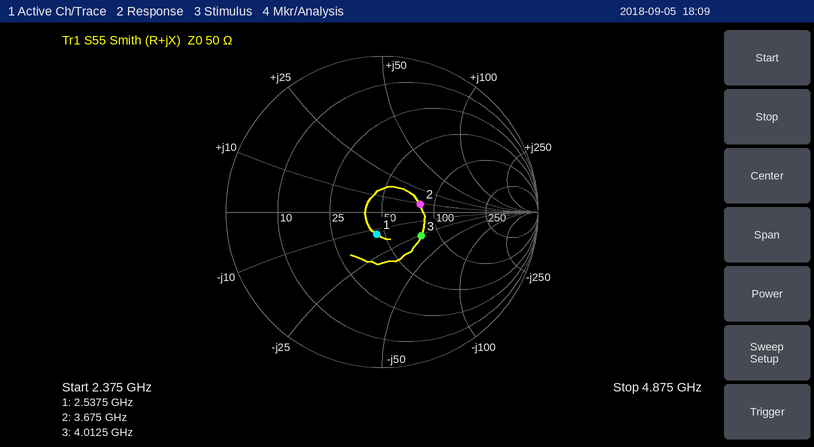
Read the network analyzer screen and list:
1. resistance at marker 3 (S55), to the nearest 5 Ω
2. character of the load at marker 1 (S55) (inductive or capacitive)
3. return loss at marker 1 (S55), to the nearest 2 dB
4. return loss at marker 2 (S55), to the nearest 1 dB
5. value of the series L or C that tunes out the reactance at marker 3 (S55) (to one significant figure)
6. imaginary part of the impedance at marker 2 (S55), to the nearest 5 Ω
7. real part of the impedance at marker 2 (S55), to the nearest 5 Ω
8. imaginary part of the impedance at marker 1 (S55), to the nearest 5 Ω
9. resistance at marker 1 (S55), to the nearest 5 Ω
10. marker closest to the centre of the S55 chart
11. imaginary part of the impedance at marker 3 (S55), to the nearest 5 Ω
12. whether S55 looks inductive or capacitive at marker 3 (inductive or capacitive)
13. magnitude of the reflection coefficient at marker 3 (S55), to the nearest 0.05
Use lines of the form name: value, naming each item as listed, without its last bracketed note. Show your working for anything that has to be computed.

resistance at marker 3 (S55), to the nearest 5 Ω: 80 Ω
character of the load at marker 1 (S55): capacitive
return loss at marker 1 (S55), to the nearest 2 dB: 16 dB
return loss at marker 2 (S55), to the nearest 1 dB: 12 dB
value of the series L or C that tunes out the reactance at marker 3 (S55): L = 25 Ω/(2π × 4.0125 GHz) ≈ 1 nH
imaginary part of the impedance at marker 2 (S55), to the nearest 5 Ω: +10 Ω
real part of the impedance at marker 2 (S55), to the nearest 5 Ω: 80 Ω
imaginary part of the impedance at marker 1 (S55), to the nearest 5 Ω: -15 Ω
resistance at marker 1 (S55), to the nearest 5 Ω: 45 Ω
marker closest to the centre of the S55 chart: marker 1
imaginary part of the impedance at marker 3 (S55), to the nearest 5 Ω: -25 Ω
whether S55 looks inductive or capacitive at marker 3: capacitive
magnitude of the reflection coefficient at marker 3 (S55), to the nearest 0.05: 0.30
